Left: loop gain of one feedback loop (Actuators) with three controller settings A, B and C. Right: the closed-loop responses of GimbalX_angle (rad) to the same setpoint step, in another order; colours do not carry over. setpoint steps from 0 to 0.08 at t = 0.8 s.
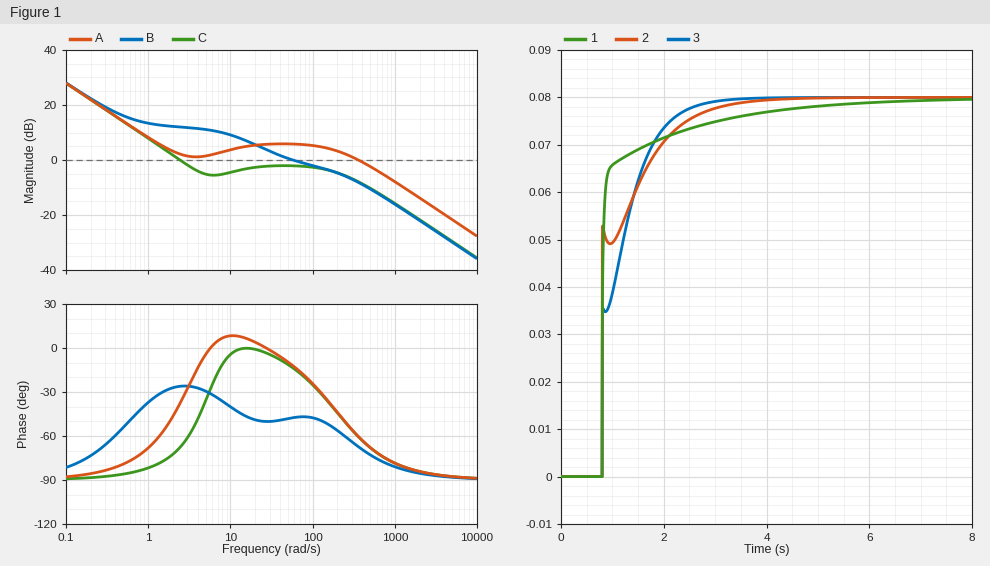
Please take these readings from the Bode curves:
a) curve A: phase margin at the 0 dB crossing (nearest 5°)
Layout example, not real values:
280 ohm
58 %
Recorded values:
120°
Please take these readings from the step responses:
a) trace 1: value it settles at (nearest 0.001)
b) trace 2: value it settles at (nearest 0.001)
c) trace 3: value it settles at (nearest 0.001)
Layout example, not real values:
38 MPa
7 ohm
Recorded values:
0.080
0.080
0.080
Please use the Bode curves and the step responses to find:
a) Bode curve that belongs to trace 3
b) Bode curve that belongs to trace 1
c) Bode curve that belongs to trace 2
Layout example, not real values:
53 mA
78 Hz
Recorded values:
C
B
A
